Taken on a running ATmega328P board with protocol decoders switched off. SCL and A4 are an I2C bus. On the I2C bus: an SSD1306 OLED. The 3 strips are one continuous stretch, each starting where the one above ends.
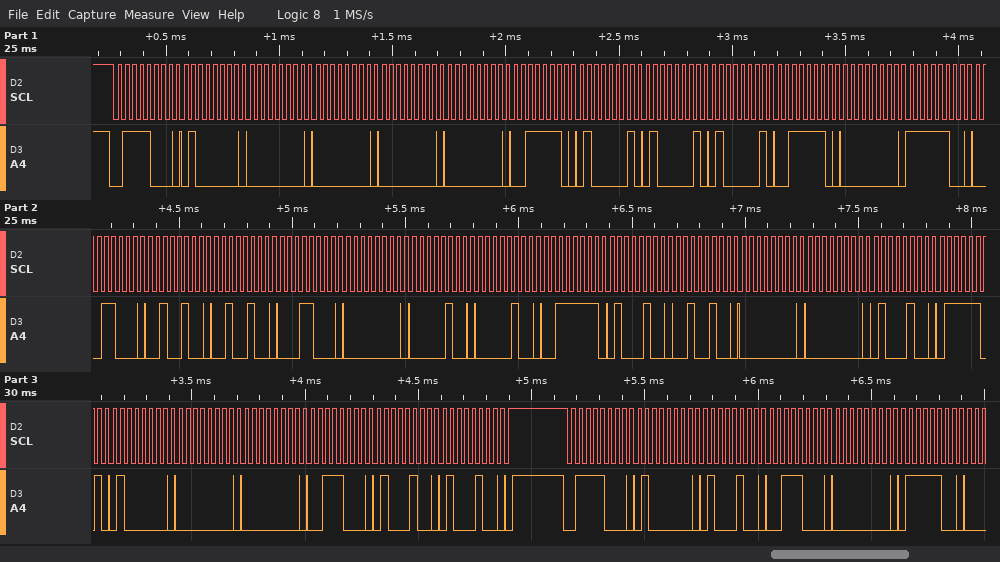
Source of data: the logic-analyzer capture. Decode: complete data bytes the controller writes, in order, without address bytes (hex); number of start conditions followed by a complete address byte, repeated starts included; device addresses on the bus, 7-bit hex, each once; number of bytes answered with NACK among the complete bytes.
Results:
40 00 00 00 00 3E 41 41 41 3E 00 FC 18 24 24 18 00 04 04 3F 44 24 00 00 44 7D 40 00 00 38 44 44 40 44 38 00 7C
2
0x3C
0
